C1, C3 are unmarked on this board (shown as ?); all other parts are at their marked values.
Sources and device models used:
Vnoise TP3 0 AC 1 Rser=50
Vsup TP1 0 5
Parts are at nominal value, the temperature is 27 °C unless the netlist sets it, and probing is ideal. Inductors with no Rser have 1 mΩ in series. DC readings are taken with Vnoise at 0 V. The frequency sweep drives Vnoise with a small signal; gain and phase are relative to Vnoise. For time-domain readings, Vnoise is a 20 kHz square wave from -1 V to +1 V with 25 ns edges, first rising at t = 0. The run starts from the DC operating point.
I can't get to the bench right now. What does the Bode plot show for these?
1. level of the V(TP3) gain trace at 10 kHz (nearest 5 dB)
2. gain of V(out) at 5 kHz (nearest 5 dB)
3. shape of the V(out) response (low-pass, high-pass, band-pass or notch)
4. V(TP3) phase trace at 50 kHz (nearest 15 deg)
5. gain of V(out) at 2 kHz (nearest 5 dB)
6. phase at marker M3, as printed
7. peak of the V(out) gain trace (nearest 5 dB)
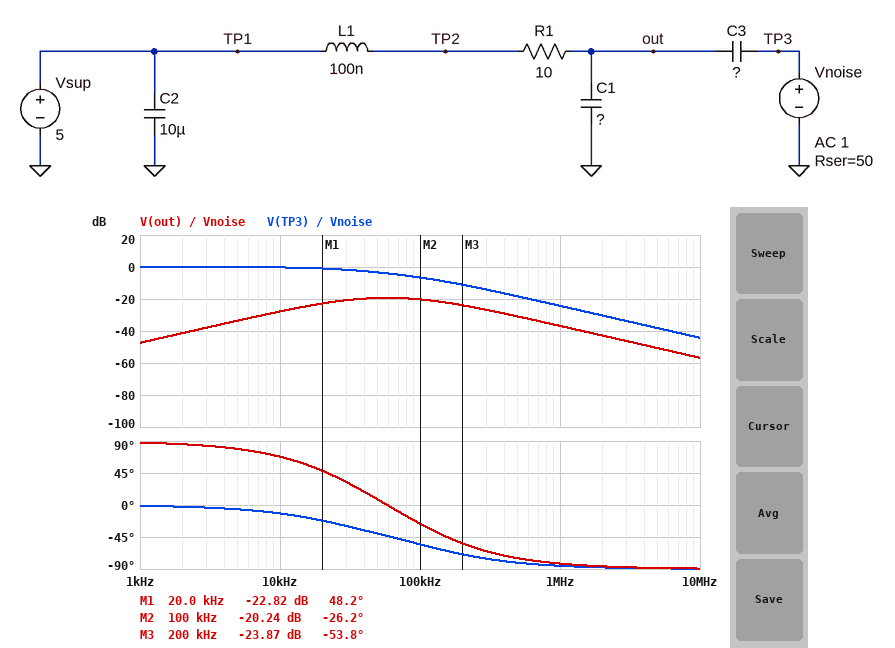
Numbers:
0 dB
-35 dB
band-pass
-45 deg
-40 dB
-53.8 deg
-20 dB
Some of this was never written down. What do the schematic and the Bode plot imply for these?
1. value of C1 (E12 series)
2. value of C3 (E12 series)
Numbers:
220 nF
68 nF
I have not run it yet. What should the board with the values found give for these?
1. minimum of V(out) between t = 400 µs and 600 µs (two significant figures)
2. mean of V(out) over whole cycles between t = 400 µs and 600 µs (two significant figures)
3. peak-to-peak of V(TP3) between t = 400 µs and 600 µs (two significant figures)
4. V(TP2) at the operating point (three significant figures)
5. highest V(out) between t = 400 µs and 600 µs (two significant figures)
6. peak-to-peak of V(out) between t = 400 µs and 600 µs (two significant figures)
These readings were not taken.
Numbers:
4.8 V
5.0 V
2.0 V
5.00 V
5.2 V
330 mV
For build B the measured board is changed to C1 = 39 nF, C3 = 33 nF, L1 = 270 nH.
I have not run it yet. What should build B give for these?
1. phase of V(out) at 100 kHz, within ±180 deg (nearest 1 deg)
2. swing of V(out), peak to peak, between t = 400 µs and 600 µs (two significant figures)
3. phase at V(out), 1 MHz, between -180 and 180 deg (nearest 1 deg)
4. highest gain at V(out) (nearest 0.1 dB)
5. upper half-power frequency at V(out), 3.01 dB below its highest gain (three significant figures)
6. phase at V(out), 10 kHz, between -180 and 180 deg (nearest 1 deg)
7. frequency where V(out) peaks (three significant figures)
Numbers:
27 deg
470 mV
-58 deg
-17.0 dB
687 kHz
82 deg
206 kHz
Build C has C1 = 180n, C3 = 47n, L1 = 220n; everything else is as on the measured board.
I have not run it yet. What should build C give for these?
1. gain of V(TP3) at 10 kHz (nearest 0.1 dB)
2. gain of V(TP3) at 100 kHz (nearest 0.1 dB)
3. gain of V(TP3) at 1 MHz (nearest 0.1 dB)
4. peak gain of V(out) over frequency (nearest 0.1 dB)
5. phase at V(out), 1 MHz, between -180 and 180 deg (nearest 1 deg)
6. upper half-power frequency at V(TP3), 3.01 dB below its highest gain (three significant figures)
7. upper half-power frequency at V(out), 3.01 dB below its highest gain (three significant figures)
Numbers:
-0.1 dB
-4.7 dB
-21.4 dB
-19.8 dB
-80 deg
66.5 kHz
205 kHz
